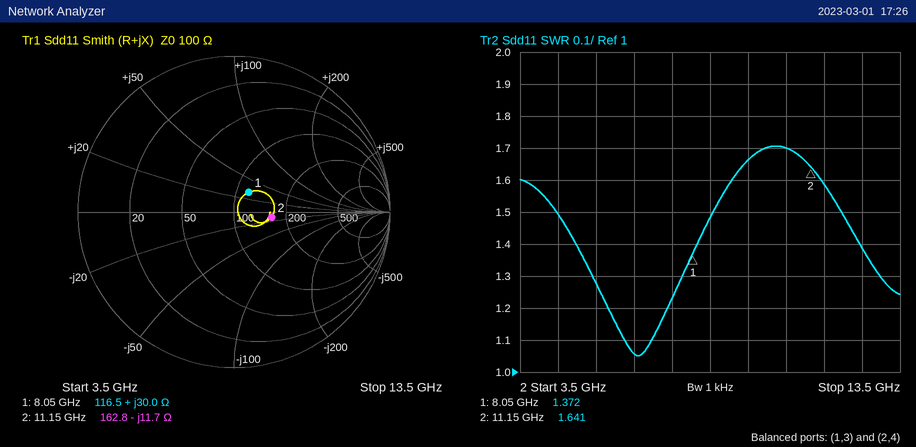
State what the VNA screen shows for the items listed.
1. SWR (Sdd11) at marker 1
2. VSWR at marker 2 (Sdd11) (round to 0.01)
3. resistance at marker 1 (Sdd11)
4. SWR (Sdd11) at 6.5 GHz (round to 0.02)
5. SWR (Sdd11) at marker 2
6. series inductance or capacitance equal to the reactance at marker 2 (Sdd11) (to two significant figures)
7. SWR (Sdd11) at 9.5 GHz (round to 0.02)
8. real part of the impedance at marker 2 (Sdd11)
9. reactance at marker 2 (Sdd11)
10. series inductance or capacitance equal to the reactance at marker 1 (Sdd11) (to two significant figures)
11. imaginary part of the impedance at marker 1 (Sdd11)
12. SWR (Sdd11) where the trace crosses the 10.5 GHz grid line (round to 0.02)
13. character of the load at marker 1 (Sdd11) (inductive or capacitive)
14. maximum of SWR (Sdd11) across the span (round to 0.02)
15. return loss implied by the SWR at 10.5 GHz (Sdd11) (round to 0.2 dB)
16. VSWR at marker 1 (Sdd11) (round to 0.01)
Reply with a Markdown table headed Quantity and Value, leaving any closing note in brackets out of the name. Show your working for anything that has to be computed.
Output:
| Quantity | Value |
|---|---|
| SWR (Sdd11) at marker 1 | 1.372 |
| VSWR at marker 2 (Sdd11) | 1.64 |
| resistance at marker 1 | 116.5 Ω |
| SWR (Sdd11) at 6.5 GHz | 1.06 |
| SWR (Sdd11) at marker 2 | 1.641 |
| series inductance or capacitance equal to the reactance at marker 2 (Sdd11) | C = 1/(2π × 11.15 GHz × 11.7 Ω) ≈ 1.2 pF |
| SWR (Sdd11) at 9.5 GHz | 1.66 |
| real part of the impedance at marker 2 | 162.8 Ω |
| reactance at marker 2 | -11.7 Ω |
| series inductance or capacitance equal to the reactance at marker 1 (Sdd11) | L = 30 Ω/(2π × 8.05 GHz) ≈ 593 pH, so 590 pH to two significant figures |
| imaginary part of the impedance at marker 1 | +30.0 Ω |
| SWR (Sdd11) where the trace crosses the 10.5 GHz grid line | 1.70 |
| character of the load at marker 1 (Sdd11) | inductive |
| maximum of SWR (Sdd11) across the span | 1.70 |
| return loss implied by the SWR at 10.5 GHz (Sdd11) | −20 log10((1.7 − 1)/(1.7 + 1)) ≈ 11.7 dB, so 11.8 dB to the nearest 0.2 dB |
| VSWR at marker 1 (Sdd11) | 1.37 |
